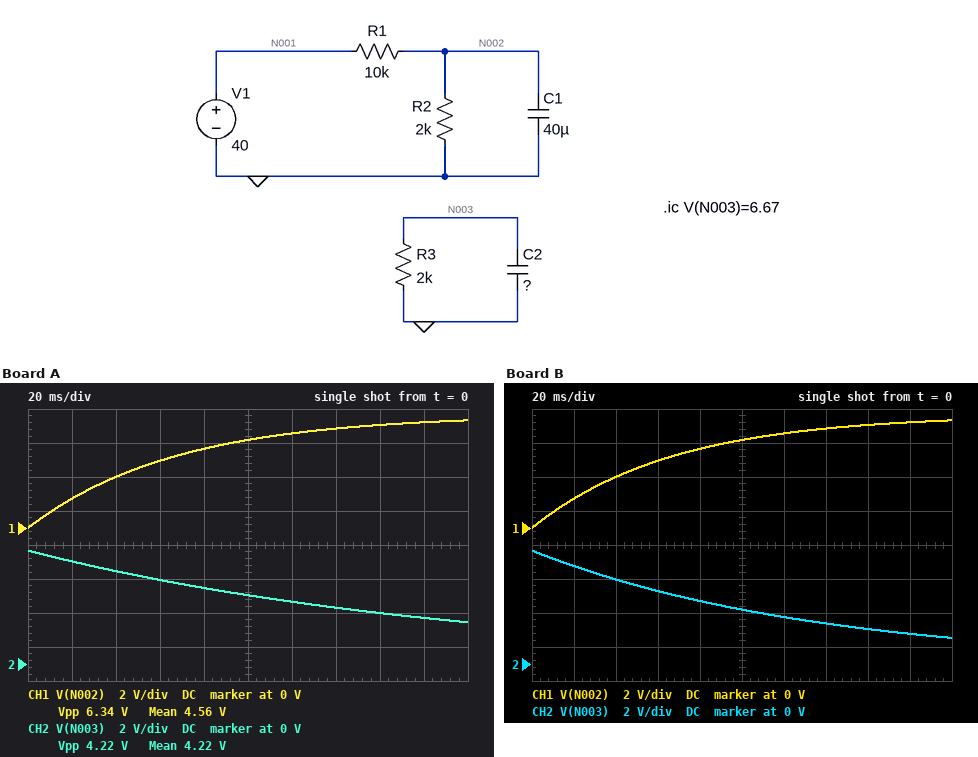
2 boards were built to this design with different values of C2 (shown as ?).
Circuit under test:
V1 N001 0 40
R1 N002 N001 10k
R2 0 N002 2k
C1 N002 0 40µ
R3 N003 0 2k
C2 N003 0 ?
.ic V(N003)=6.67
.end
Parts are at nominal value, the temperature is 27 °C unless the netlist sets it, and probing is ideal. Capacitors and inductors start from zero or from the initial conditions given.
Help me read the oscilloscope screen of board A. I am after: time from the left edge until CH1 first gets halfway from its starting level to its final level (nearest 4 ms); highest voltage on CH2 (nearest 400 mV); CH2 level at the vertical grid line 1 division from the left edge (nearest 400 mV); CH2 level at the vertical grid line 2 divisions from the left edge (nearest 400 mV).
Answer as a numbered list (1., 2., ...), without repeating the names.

1. 44 ms
2. 6.8 V
3. 6.0 V
4. 5.6 V
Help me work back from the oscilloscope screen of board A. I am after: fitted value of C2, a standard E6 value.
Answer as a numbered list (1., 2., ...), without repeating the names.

1. 100 µF
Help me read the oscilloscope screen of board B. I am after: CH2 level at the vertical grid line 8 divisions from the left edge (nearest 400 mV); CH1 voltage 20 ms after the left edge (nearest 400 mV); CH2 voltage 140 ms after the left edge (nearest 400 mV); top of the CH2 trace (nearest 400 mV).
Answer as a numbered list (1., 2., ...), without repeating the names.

1. 2.0 V
2. 1.6 V
3. 2.4 V
4. 6.8 V
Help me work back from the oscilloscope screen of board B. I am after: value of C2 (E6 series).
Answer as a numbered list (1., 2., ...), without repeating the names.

1. 68 µF
